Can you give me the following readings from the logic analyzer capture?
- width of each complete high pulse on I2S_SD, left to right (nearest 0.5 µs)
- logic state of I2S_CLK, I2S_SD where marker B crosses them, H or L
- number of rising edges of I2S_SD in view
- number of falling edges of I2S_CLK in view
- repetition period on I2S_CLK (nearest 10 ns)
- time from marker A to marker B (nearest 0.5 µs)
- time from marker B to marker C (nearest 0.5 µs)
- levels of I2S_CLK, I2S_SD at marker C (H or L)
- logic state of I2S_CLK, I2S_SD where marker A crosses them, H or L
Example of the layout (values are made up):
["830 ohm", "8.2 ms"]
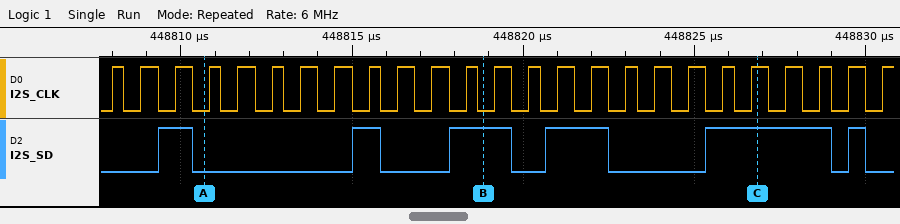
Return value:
["1 µs, 1 µs, 2 µs, 2 µs, 3.5 µs, 0.5 µs", "I2S_CLK=L, I2S_SD=H", "6", "24", "940 ns", "8 µs", "8 µs", "I2S_CLK=H, I2S_SD=H", "I2S_CLK=L, I2S_SD=L"]
